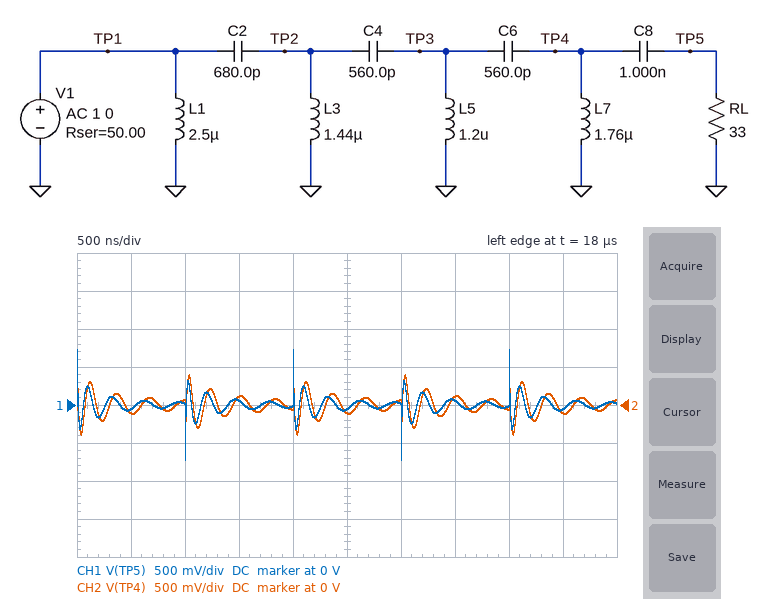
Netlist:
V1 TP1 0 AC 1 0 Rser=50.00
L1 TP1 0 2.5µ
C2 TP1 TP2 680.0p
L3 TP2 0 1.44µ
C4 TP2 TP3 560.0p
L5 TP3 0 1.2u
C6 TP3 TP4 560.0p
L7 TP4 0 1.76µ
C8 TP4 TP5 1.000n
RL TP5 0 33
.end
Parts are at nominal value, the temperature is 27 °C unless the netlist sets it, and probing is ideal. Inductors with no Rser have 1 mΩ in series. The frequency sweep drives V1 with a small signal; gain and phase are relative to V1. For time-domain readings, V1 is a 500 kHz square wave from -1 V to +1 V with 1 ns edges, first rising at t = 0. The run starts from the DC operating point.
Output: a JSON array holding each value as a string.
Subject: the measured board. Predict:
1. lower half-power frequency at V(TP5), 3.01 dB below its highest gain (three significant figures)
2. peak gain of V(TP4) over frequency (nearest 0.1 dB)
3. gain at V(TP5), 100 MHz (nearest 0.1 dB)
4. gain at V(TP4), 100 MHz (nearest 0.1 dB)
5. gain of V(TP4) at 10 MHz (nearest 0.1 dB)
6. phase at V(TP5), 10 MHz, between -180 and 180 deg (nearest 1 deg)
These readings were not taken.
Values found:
["2.95 MHz", "-3.3 dB", "-8.0 dB", "-8.0 dB", "-7.2 dB", "115 deg"]
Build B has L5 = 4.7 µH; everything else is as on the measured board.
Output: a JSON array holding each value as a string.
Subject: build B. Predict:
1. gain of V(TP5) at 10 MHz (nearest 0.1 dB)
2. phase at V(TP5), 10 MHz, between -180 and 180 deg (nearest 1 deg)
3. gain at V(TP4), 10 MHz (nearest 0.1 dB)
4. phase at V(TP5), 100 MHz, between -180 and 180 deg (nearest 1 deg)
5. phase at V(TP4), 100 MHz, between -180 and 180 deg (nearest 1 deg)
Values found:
["-8.7 dB", "100 deg", "-7.8 dB", "10 deg", "7 deg"]
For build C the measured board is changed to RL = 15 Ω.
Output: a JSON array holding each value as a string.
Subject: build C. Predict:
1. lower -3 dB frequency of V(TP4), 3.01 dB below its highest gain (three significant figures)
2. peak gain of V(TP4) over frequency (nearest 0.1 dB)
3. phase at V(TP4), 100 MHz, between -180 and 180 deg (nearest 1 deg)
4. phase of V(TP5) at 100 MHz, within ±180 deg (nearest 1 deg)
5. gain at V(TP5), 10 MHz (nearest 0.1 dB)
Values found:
["2.79 MHz", "-2.2 dB", "5 deg", "11 deg", "-12.8 dB"]
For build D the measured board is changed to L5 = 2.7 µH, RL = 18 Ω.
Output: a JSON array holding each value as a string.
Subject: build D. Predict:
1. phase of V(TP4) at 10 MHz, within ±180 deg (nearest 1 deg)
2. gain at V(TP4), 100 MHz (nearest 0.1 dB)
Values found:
["64 deg", "-11.5 dB"]
